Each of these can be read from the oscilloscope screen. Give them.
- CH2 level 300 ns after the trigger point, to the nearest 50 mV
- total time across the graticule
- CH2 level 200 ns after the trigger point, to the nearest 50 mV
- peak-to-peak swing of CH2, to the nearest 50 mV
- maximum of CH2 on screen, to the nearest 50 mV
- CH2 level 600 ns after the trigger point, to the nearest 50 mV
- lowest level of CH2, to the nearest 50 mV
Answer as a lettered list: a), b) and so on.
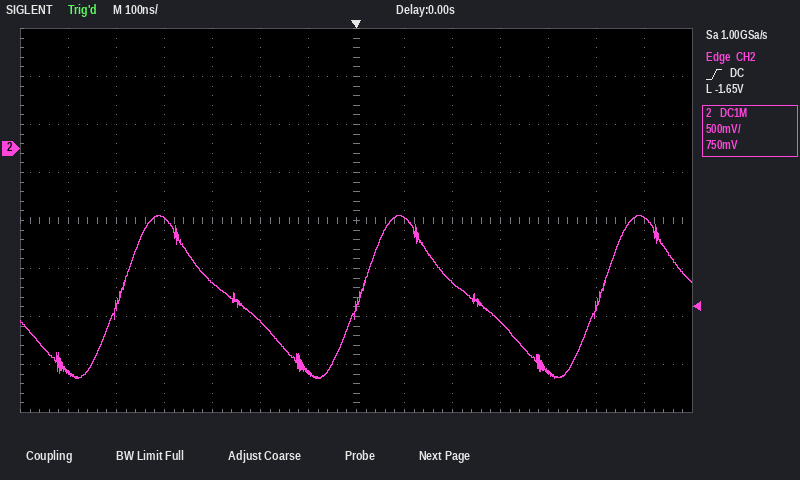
a) -1.80 V
b) 1.4 µs
c) -1.40 V
d) 1.70 V
e) -700 mV
f) -700 mV
g) -2.40 V
